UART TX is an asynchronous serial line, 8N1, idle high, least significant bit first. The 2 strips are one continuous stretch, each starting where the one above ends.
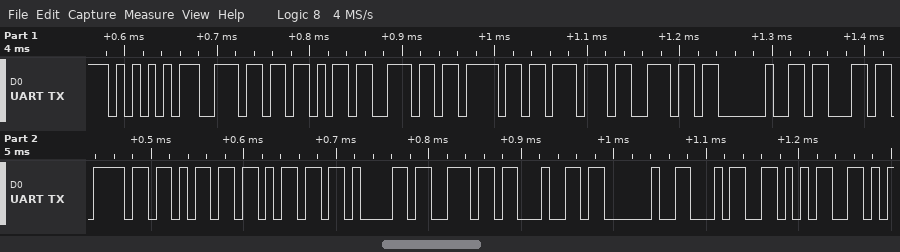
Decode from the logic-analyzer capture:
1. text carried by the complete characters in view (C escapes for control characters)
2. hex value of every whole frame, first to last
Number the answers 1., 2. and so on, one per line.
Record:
1. "Unknown command 45"
2. 55 6E 6B 6E 6F 77 6E 20 63 6F 6D 6D 61 6E 64 20 34 35
